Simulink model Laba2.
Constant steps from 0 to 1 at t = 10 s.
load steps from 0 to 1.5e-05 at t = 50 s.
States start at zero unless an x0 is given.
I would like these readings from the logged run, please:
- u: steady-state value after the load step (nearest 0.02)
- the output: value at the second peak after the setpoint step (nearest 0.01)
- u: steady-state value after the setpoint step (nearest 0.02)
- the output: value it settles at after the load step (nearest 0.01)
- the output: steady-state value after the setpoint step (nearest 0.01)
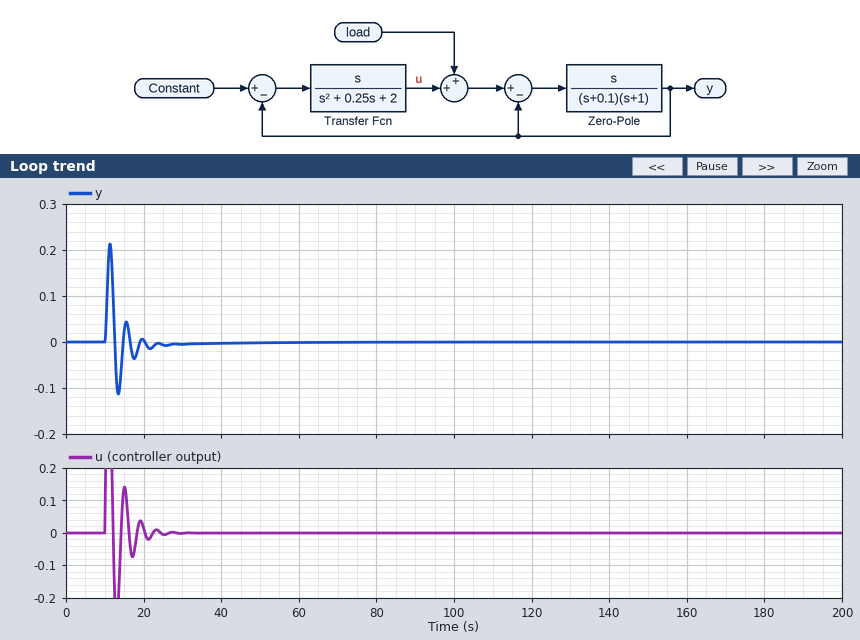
0.00
0.04
0.00
0.00
0.00
